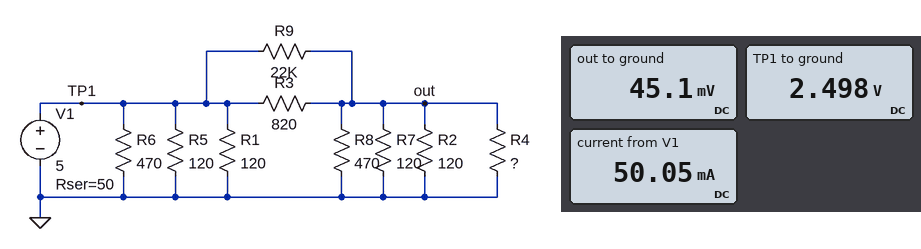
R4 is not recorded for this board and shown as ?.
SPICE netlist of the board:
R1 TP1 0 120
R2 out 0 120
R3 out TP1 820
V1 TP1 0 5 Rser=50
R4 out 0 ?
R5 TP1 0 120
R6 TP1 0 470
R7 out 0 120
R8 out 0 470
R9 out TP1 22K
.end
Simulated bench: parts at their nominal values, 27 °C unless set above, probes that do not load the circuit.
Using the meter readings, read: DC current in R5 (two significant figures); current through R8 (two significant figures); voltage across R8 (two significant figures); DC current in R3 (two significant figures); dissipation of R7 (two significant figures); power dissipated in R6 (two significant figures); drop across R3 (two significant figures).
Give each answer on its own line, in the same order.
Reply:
21 mA
96 µA
45 mV
3.0 mA
17 µW
13 mW
2.5 V
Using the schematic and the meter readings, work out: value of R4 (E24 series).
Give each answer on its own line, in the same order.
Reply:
20 Ω
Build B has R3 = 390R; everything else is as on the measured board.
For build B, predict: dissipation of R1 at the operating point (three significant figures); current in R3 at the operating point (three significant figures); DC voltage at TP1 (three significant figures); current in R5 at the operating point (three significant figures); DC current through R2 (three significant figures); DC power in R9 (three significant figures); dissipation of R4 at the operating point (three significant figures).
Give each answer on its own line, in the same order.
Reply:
48.8 mW
5.98 mA
2.42 V
20.2 mA
737 µA
247 µW
391 µW
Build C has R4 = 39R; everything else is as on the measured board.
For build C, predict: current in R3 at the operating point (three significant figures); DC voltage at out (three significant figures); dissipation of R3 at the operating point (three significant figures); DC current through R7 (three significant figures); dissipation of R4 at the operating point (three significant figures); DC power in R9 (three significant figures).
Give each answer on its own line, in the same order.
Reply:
2.96 mA
69.2 mV
7.20 mW
576 µA
123 µW
268 µW
